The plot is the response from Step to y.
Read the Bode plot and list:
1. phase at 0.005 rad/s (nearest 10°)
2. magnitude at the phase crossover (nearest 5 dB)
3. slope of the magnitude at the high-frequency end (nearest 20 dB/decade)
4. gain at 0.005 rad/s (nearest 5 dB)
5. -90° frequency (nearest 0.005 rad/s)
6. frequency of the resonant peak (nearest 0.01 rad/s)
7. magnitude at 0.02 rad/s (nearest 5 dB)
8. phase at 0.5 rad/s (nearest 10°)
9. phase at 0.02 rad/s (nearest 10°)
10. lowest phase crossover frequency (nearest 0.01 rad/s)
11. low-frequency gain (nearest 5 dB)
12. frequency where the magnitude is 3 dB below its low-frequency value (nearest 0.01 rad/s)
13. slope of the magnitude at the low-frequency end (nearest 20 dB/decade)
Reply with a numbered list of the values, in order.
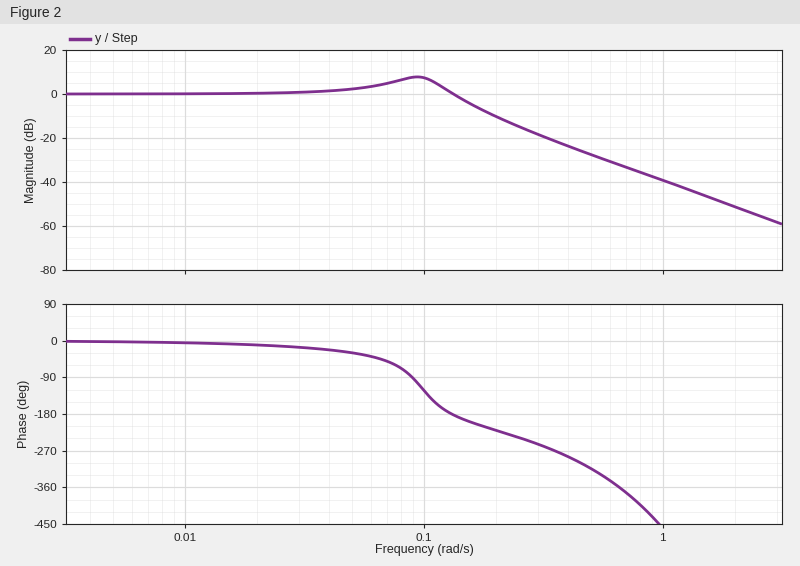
1. 0°
2. 0 dB
3. -40 dB/decade
4. 0 dB
5. 0.090 rad/s
6. 0.09 rad/s
7. 0 dB
8. -310°
9. -10°
10. 0.13 rad/s
11. 0 dB
12. 0.15 rad/s
13. 0 dB/decade
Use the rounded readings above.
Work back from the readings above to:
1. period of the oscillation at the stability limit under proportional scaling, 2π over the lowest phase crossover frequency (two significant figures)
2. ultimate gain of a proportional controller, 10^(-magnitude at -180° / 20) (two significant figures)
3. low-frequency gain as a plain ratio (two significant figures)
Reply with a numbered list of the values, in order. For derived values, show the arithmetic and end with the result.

1. 2π / 0.13 = 48 s
2. 10^(0 / 20) = 1.0
3. 10^(0 / 20) = 1.0
